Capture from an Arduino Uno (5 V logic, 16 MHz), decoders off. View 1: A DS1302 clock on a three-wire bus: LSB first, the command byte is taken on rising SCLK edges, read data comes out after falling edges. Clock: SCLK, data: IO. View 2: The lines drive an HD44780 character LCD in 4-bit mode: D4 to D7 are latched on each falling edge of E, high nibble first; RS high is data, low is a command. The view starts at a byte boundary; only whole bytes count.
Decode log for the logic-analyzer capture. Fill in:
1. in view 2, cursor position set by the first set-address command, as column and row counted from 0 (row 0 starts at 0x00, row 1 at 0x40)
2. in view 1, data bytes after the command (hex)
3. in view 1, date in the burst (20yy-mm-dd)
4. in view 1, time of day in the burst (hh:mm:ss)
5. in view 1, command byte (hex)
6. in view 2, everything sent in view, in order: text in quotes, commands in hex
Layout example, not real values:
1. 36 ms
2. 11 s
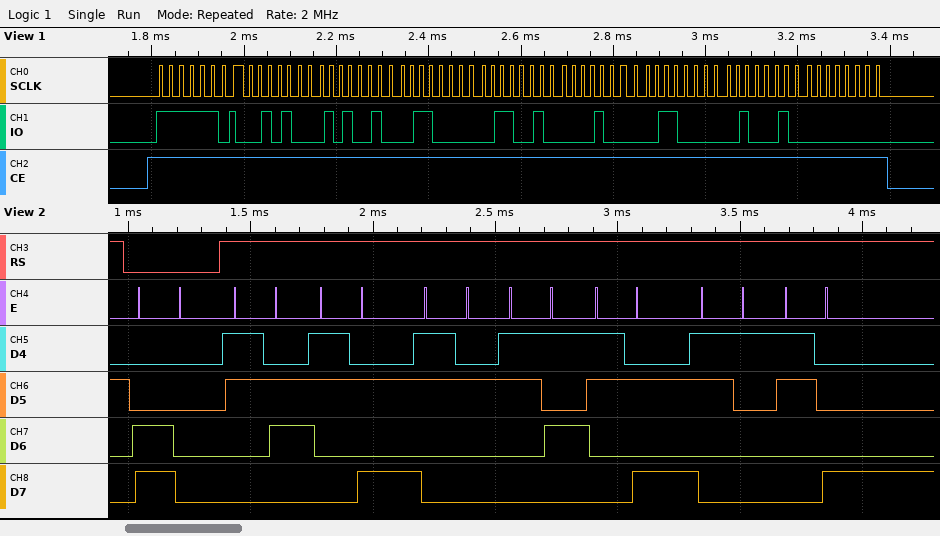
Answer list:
1. column 0, row 1
2. 14 25 06 26 08 06 22 00
3. 2022-08-26
4. 06:25:14
5. 0xBF
6. 0xC0 "6:25:18"
